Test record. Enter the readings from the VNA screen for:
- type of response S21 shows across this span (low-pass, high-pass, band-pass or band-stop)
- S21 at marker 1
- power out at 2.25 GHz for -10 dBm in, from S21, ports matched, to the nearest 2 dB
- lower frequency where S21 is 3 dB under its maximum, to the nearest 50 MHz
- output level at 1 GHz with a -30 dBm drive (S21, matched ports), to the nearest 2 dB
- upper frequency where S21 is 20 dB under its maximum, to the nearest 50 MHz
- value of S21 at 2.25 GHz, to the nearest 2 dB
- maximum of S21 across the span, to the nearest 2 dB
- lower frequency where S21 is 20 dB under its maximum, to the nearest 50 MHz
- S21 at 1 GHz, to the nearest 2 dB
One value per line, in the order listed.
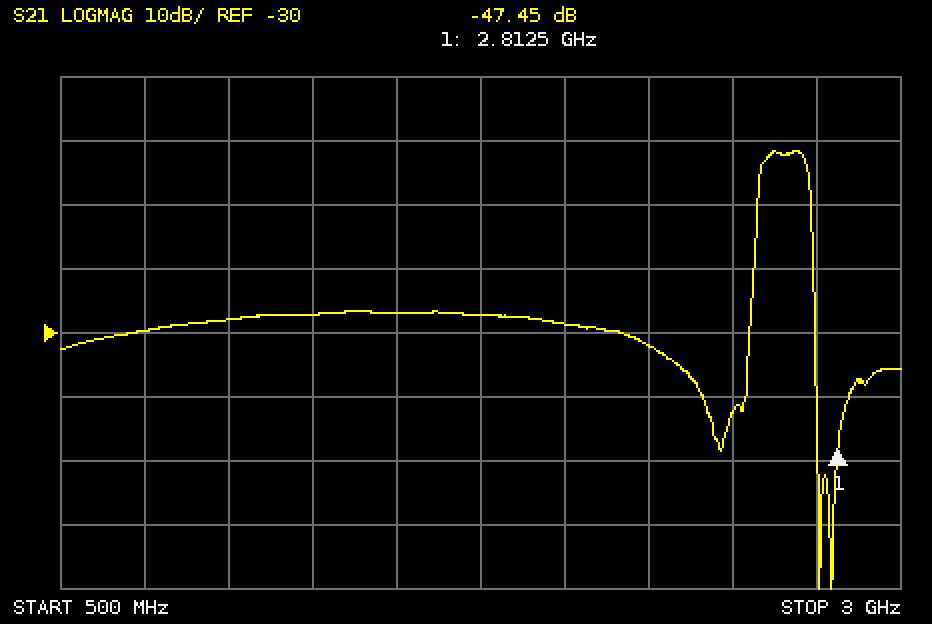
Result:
band-pass
-47.45 dB
-42 dBm
2.60 GHz
-58 dBm
2.75 GHz
-32 dB
-2 dB
2.55 GHz
-28 dB
